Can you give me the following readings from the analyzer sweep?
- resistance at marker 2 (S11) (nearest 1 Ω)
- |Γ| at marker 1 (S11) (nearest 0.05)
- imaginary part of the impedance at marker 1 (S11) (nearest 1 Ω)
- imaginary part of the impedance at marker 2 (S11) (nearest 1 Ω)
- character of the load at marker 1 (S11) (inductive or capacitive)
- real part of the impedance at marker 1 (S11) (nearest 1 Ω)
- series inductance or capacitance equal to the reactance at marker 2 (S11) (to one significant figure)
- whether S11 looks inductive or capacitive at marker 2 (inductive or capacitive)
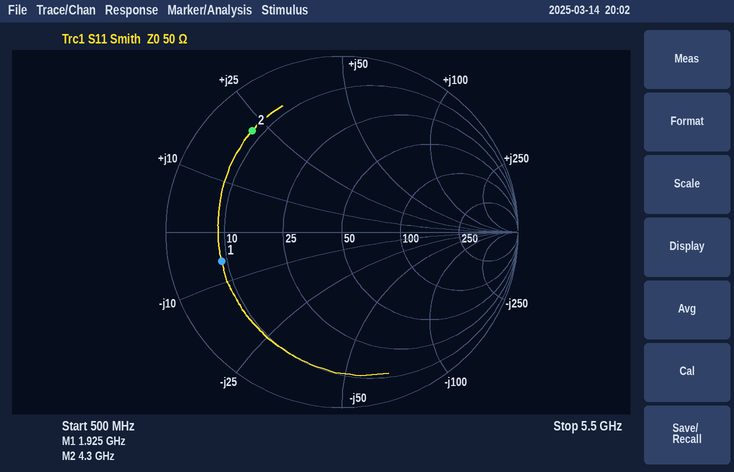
8 Ω
0.70
-6 Ω
+22 Ω
capacitive
9 Ω
800 pH
inductive
